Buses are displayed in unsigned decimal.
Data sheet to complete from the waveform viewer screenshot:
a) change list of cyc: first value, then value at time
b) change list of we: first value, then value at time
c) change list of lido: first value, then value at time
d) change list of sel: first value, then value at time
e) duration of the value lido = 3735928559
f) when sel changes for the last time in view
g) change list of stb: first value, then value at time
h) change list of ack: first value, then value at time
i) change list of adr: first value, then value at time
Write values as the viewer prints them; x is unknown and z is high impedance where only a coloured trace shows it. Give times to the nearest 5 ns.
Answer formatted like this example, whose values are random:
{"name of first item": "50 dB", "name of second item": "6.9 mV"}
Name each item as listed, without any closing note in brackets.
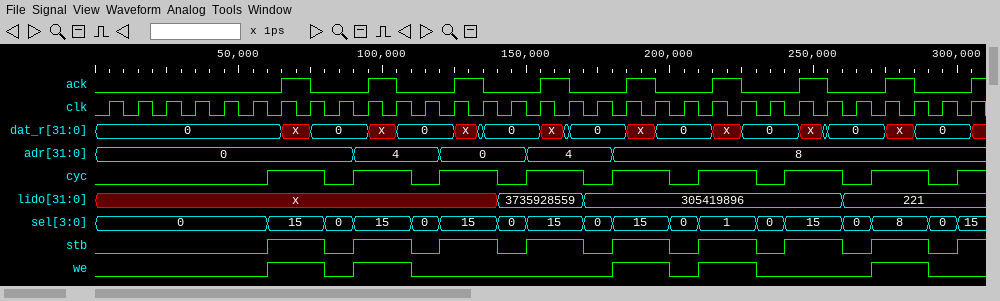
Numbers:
{"change list of cyc: first value, then value at time": "0, 1 at 60 ns, 0 at 80 ns, 1 at 90 ns, 0 at 110 ns, 1 at 120 ns, 0 at 140 ns, 1 at 150 ns, 0 at 170 ns, 1 at 180 ns, 0 at 200 ns, 1 at 210 ns, 0 at 230 ns, 1 at 240 ns, 0 at 260 ns, 1 at 270 ns, 0 at 290 ns, 1 at 300 ns", "change list of we: first value, then value at time": "0, 1 at 60 ns, 0 at 80 ns, 1 at 90 ns, 0 at 110 ns, 1 at 180 ns, 0 at 200 ns, 1 at 210 ns, 0 at 230 ns, 1 at 270 ns, 0 at 290 ns", "change list of lido: first value, then value at time": "x, 3735928559 at 140 ns, 305419896 at 170 ns, 221 at 260 ns", "change list of sel: first value, then value at time": "0, 15 at 60 ns, 0 at 80 ns, 15 at 90 ns, 0 at 110 ns, 15 at 120 ns, 0 at 140 ns, 15 at 150 ns, 0 at 170 ns, 15 at 180 ns, 0 at 200 ns, 1 at 210 ns, 0 at 230 ns, 15 at 240 ns, 0 at 260 ns, 8 at 270 ns, 0 at 290 ns, 15 at 300 ns", "duration of the value lido = 3735928559": "30 ns", "when sel changes for the last time in view": "300 ns", "change list of stb: first value, then value at time": "0, 1 at 60 ns, 0 at 80 ns, 1 at 90 ns, 0 at 110 ns, 1 at 120 ns, 0 at 140 ns, 1 at 150 ns, 0 at 170 ns, 1 at 180 ns, 0 at 200 ns, 1 at 210 ns, 0 at 230 ns, 1 at 240 ns, 0 at 260 ns, 1 at 270 ns, 0 at 290 ns, 1 at 300 ns", "change list of ack: first value, then value at time": "0, 1 at 65 ns, 0 at 75 ns, 1 at 95 ns, 0 at 105 ns, 1 at 125 ns, 0 at 135 ns, 1 at 155 ns, 0 at 165 ns, 1 at 185 ns, 0 at 195 ns, 1 at 215 ns, 0 at 225 ns, 1 at 245 ns, 0 at 255 ns, 1 at 275 ns, 0 at 285 ns, 1 at 305 ns", "change list of adr: first value, then value at time": "0, 4 at 90 ns, 0 at 120 ns, 4 at 150 ns, 8 at 180 ns"}
